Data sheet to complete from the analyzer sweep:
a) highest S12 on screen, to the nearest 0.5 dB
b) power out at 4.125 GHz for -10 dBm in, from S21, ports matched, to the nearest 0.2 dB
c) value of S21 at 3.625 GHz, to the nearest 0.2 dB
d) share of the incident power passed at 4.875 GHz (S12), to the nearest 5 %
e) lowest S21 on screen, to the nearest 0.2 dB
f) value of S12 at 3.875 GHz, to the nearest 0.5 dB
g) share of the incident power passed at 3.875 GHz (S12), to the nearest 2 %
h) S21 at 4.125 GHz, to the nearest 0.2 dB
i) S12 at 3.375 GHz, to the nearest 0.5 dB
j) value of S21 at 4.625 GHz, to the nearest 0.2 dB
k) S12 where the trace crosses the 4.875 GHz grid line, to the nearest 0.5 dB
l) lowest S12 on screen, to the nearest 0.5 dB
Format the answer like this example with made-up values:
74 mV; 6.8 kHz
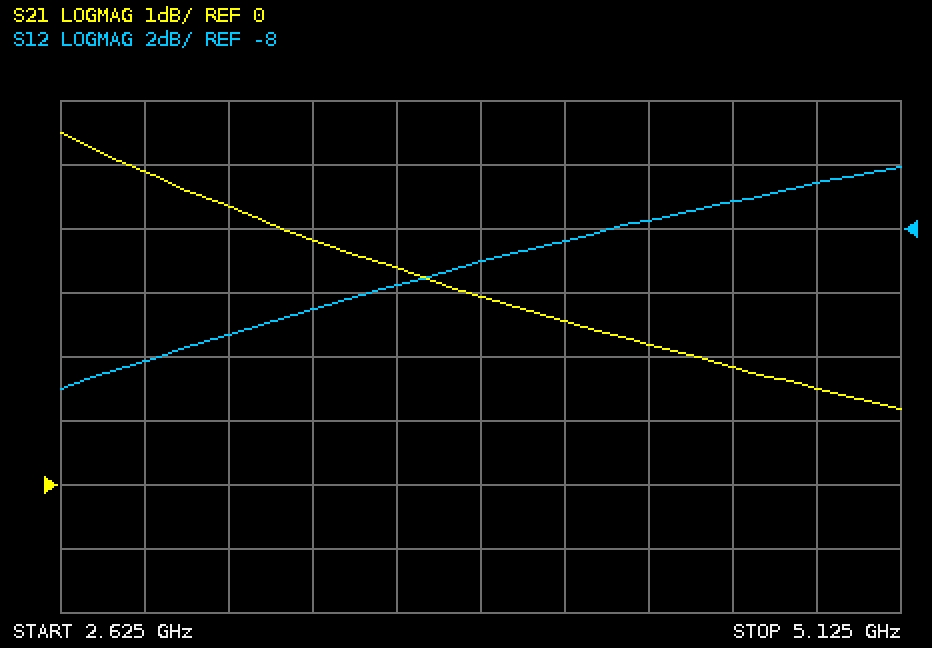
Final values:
-6.0 dB; -7.4 dBm; 3.4 dB; 20 %; 1.2 dB; -9.0 dB; 12 %; 2.6 dB; -10.5 dB; 1.8 dB; -6.5 dB; -13.0 dB
